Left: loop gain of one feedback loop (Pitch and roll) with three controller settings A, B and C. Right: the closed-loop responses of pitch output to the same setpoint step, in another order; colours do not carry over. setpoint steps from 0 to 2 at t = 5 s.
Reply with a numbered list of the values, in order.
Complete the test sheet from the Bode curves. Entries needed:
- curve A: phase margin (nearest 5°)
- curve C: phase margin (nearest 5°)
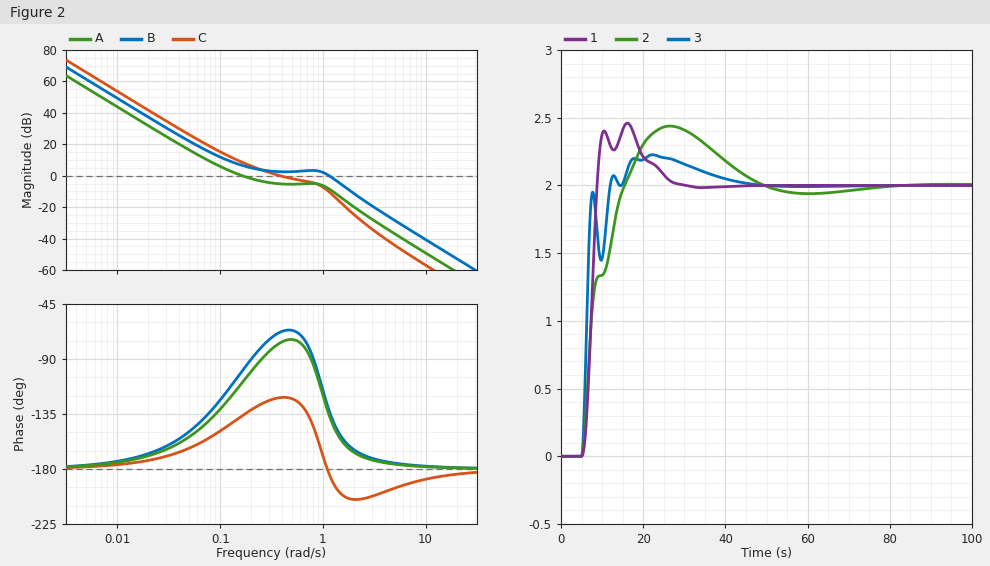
1. 70°
2. 60°
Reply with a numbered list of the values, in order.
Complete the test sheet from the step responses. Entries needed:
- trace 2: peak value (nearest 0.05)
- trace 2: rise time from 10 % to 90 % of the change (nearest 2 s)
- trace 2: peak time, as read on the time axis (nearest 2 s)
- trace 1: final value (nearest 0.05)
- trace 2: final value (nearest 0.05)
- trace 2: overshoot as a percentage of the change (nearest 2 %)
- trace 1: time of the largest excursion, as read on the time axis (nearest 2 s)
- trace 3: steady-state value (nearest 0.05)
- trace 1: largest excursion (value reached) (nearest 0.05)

1. 2.45
2. 8 s
3. 26 s
4. 2.00
5. 2.00
6. 22 %
7. 16 s
8. 2.00
9. 2.45
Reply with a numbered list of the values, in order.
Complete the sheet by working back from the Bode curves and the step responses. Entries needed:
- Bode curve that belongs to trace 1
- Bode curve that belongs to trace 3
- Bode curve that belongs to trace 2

1. C
2. B
3. A
